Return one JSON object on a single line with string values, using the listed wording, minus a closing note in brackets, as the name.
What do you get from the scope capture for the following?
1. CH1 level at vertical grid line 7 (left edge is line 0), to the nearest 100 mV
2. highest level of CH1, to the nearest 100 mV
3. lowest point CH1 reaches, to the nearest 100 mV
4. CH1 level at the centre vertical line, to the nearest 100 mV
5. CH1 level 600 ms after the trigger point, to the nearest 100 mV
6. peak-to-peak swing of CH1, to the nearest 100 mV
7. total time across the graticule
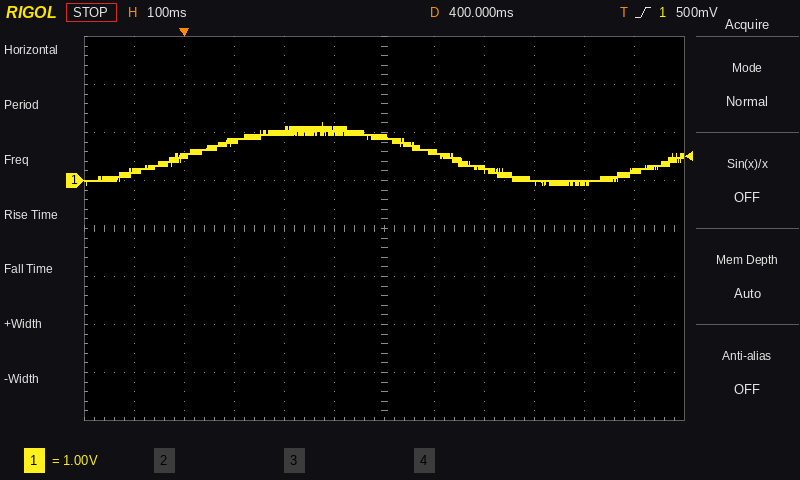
{"CH1 level at vertical grid line 7 (left edge is line 0), to the nearest 100 mV": "600 mV", "highest level of CH1, to the nearest 100 mV": "1.2 V", "lowest point CH1 reaches, to the nearest 100 mV": "-100 mV", "CH1 level at the centre vertical line, to the nearest 100 mV": "900 mV", "CH1 level 600 ms after the trigger point, to the nearest 100 mV": "200 mV", "peak-to-peak swing of CH1, to the nearest 100 mV": "1.3 V", "total time across the graticule": "1.2 s"}
